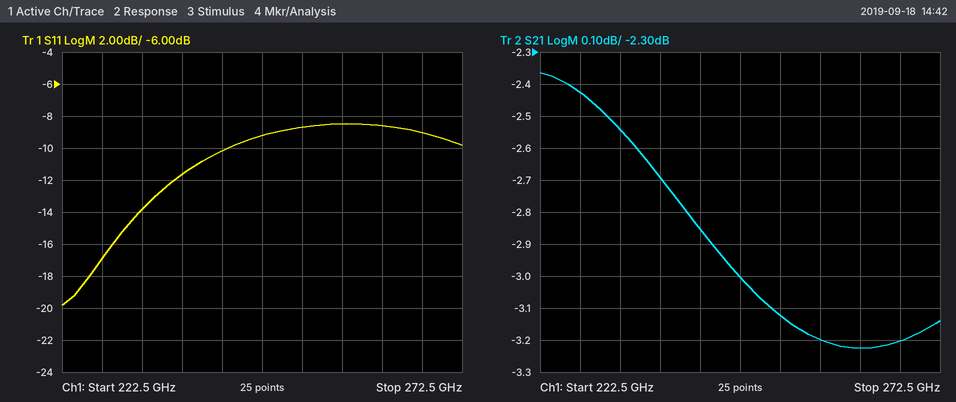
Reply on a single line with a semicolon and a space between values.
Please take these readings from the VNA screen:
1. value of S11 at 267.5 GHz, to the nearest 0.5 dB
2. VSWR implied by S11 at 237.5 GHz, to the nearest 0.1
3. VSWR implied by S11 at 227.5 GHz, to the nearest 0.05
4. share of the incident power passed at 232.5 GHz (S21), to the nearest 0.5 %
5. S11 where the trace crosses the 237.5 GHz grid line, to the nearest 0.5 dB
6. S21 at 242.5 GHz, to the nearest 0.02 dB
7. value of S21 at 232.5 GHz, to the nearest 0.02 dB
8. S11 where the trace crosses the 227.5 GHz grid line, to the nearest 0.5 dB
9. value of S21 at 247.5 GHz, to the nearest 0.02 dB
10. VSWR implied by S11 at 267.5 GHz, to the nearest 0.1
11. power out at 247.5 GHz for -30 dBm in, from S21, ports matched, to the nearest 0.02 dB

-9.0 dB; 1.7; 1.35; 55.5 %; -11.5 dB; -2.86 dB; -2.54 dB; -17.0 dB; -3.00 dB; 2.1; -33.00 dBm
